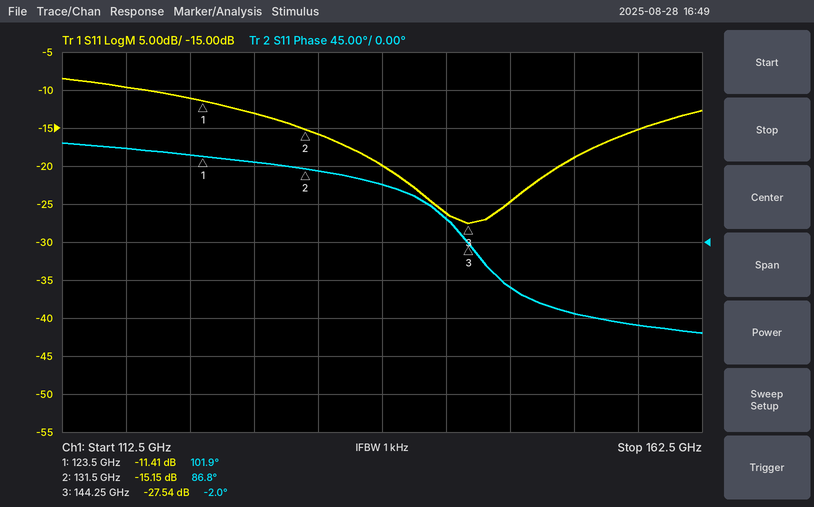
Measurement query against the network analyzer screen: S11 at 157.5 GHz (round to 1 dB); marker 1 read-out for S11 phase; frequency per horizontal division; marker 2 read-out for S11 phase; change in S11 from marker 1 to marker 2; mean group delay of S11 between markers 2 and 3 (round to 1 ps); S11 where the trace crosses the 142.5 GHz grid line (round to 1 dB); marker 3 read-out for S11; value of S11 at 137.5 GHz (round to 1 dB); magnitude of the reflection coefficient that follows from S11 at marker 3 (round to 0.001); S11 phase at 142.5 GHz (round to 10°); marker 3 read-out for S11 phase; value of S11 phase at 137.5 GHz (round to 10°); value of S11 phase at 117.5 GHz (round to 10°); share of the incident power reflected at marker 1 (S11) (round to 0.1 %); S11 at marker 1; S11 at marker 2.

-15 dB
101.9°
5 GHz
86.8°
-3.74 dB
19 ps
-26 dB
-27.54 dB
-20 dB
0.042
30°
-2.0°
70°
110°
7.2 %
-11.41 dB
-15.15 dB
